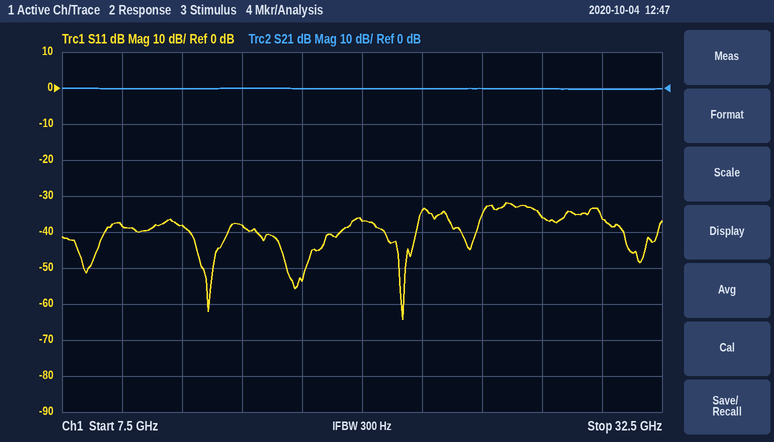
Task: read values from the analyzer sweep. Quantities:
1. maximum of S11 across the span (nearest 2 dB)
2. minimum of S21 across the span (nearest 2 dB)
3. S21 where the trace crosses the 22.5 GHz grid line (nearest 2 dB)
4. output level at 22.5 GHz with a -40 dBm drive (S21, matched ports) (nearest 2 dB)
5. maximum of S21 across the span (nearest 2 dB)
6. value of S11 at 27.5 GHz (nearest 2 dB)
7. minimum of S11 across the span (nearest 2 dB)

-32 dB
0 dB
0 dB
-40 dBm
0 dB
-36 dB
-64 dB
